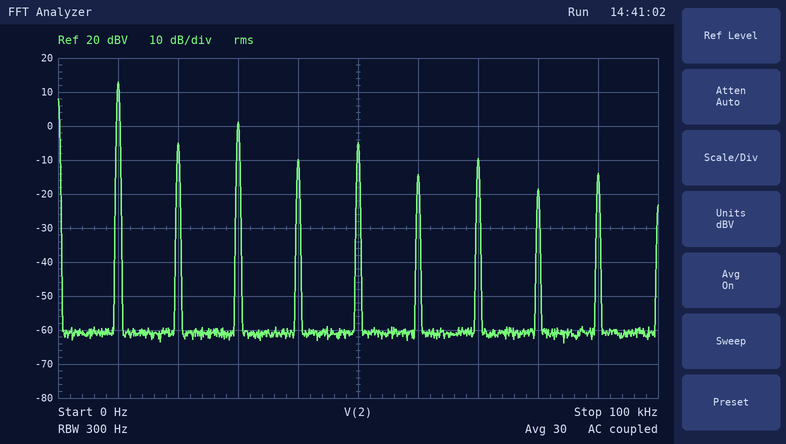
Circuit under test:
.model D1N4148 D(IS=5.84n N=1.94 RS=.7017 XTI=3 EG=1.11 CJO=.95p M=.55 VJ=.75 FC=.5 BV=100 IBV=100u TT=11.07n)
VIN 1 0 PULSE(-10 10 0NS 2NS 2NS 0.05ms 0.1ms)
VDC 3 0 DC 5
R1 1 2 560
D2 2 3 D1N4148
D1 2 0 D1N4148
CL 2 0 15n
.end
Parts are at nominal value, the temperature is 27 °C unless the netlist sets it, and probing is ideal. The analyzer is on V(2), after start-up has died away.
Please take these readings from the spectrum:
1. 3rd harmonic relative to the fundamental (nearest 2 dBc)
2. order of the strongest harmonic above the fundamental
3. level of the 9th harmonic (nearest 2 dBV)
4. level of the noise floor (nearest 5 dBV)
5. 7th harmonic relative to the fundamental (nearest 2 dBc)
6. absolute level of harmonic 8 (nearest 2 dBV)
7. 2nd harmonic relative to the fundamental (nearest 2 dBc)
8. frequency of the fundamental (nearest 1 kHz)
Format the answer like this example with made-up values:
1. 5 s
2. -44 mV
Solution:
1. -12 dBc
2. 3
3. -14 dBV
4. -60 dBV
5. -22 dBc
6. -18 dBV
7. -18 dBc
8. 10 kHz
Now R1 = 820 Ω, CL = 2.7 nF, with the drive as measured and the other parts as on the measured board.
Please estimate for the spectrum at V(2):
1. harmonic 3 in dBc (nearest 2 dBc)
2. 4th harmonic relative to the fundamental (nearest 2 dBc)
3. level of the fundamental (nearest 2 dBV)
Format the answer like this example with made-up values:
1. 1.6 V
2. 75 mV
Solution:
1. -10 dBc
2. -28 dBc
3. 14 dBV
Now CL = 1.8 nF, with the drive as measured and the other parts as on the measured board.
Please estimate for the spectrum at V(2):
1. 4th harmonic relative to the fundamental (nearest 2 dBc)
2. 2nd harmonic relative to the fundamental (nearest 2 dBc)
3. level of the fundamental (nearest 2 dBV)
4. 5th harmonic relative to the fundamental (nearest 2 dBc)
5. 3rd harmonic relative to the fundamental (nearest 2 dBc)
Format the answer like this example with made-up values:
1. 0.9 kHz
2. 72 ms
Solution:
1. -34 dBc
2. -34 dBc
3. 14 dBV
4. -14 dBc
5. -10 dBc
